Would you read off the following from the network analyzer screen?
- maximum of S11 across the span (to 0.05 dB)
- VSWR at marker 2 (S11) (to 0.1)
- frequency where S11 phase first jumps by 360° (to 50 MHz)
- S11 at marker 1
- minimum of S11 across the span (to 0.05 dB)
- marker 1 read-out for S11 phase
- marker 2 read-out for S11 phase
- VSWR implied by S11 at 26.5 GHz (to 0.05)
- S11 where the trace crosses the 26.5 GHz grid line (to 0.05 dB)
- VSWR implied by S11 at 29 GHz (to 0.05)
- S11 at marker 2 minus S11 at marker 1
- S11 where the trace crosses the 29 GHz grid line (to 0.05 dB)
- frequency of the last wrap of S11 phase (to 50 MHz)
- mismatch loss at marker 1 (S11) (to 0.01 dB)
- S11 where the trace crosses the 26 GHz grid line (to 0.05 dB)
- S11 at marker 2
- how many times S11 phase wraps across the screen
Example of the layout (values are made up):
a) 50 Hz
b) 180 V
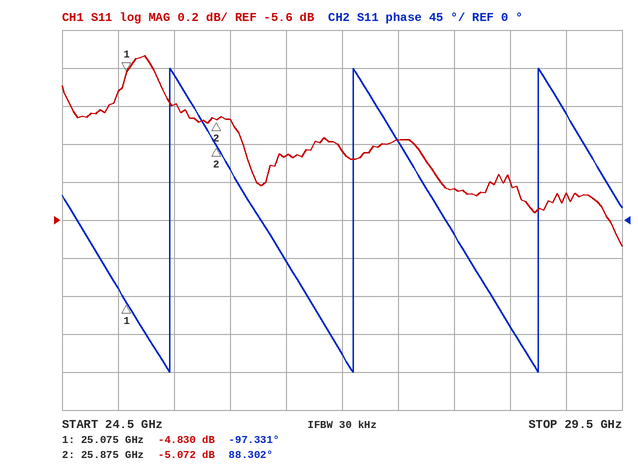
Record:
a) -4.75 dB
b) 3.5
c) 25.45 GHz
d) -4.830 dB
e) -5.75 dB
f) -97.331°
g) 88.302°
h) 3.40
i) -5.25 dB
j) 3.30
k) -0.242 dB
l) -5.45 dB
m) 28.75 GHz
n) 1.73 dB
o) -5.05 dB
p) -5.072 dB
q) 3
